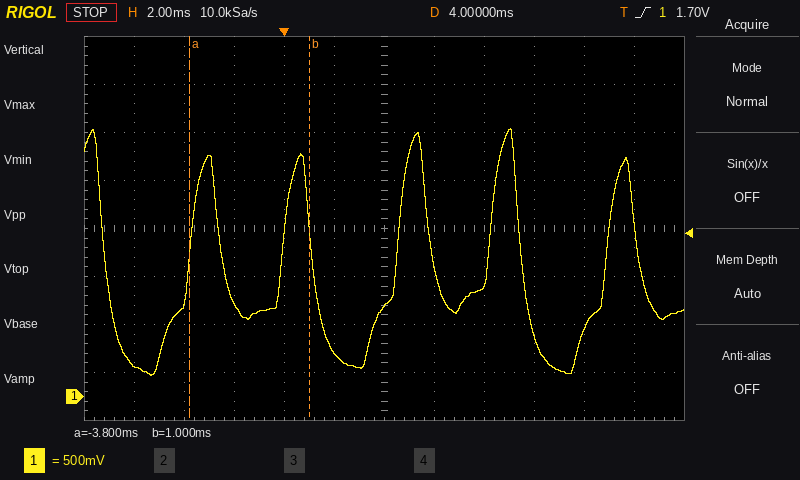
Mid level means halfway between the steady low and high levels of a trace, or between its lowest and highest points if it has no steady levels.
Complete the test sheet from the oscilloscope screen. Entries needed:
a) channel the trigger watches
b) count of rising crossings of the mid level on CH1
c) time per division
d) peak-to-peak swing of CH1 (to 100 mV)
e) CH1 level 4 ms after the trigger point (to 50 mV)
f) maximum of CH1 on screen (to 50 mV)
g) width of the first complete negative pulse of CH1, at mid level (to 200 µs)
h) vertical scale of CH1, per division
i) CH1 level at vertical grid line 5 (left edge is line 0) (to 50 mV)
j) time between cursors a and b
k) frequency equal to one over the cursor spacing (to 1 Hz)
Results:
CH1
5
2 ms
2.60 V
950 mV
2.80 V
3.4 ms
500 mV
450 mV
4.8 ms
208 Hz
